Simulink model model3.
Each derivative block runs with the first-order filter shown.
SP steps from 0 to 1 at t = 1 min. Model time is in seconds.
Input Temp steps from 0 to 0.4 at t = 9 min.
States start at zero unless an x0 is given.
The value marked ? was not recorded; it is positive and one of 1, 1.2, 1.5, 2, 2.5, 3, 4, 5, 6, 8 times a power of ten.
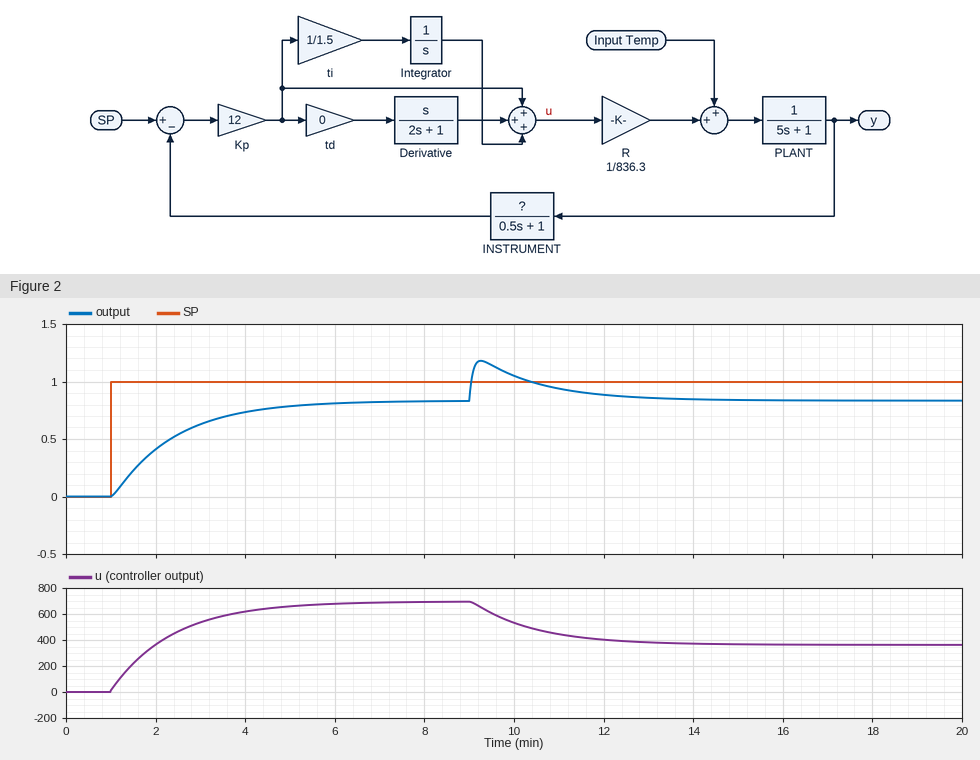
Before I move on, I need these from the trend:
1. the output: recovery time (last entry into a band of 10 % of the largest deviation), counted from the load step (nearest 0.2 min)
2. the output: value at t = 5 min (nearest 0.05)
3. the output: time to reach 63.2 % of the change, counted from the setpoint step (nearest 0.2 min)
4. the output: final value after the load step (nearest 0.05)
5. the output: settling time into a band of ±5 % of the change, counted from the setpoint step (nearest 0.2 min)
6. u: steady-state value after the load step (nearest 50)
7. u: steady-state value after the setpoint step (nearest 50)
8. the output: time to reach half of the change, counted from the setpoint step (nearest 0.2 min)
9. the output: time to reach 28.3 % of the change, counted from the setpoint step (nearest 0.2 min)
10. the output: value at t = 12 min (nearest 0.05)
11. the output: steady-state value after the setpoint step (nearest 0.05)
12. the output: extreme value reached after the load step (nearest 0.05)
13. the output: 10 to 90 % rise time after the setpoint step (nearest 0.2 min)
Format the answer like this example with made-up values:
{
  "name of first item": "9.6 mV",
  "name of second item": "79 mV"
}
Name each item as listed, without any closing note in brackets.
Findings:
{
  "the output: recovery time (last entry into a band of 10 % of the largest deviation), counted from the load step": "3.6 min",
  "the output: value at t = 5 min": "0.80",
  "the output: time to reach 63.2 % of the change, counted from the setpoint step": "1.4 min",
  "the output: final value after the load step": "0.85",
  "the output: settling time into a band of ±5 % of the change, counted from the setpoint step": "4.2 min",
  "u: steady-state value after the load step": "350",
  "u: steady-state value after the setpoint step": "700",
  "the output: time to reach half of the change, counted from the setpoint step": "1.0 min",
  "the output: time to reach 28.3 % of the change, counted from the setpoint step": "0.6 min",
  "the output: value at t = 12 min": "0.90",
  "the output: steady-state value after the setpoint step": "0.85",
  "the output: extreme value reached after the load step": "1.20",
  "the output: 10 to 90 % rise time after the setpoint step": "3.0 min"
}
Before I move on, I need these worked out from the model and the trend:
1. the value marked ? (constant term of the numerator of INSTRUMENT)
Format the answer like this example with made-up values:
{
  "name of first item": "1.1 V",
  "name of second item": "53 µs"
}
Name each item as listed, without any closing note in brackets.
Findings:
{
  "the value marked ?": "1.2"
}
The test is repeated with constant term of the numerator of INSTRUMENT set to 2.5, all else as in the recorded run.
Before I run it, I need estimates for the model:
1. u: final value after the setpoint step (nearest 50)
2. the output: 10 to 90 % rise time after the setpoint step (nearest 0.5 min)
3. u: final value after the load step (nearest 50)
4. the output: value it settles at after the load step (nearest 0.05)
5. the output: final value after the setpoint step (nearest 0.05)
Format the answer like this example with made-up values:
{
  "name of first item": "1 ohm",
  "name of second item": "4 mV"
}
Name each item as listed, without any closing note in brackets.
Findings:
{
  "u: final value after the setpoint step": "350",
  "the output: 10 to 90 % rise time after the setpoint step": "1.5 min",
  "u: final value after the load step": "0",
  "the output: value it settles at after the load step": "0.40",
  "the output: final value after the setpoint step": "0.40"
}
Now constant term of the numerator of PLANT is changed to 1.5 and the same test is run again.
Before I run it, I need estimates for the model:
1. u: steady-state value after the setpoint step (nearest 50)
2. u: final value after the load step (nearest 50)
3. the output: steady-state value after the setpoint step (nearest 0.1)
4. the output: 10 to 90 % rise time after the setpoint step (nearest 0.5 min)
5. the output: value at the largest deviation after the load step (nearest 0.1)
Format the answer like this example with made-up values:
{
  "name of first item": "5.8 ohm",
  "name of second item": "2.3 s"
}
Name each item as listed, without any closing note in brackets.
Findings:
{
  "u: steady-state value after the setpoint step": "450",
  "u: final value after the load step": "150",
  "the output: steady-state value after the setpoint step": "0.8",
  "the output: 10 to 90 % rise time after the setpoint step": "2.0 min",
  "the output: value at the largest deviation after the load step": "1.3"
}
